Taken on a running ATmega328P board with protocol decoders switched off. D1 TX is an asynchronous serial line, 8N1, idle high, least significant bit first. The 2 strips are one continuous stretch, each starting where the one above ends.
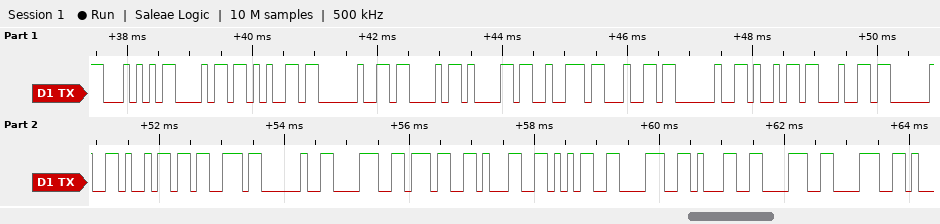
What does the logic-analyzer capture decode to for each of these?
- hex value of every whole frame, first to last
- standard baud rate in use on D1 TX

54 68 65 20 43 61 72 64 20 69 64 20 69 73 20 38 37 31 35 38 31 38 38
9600 baud
